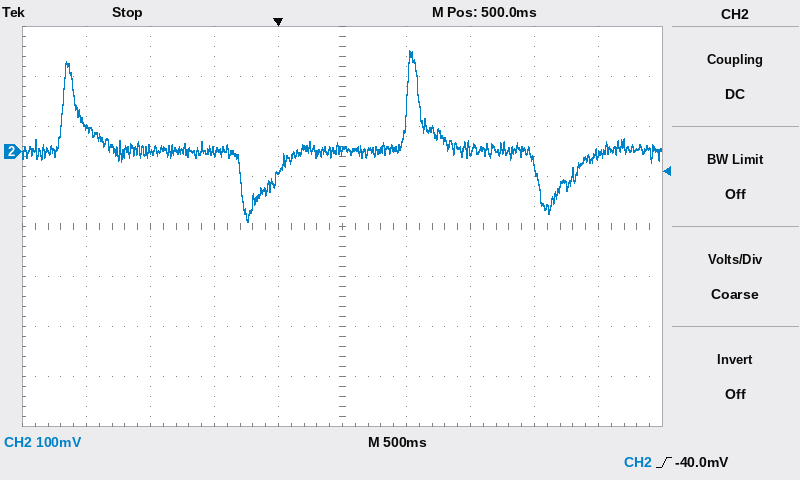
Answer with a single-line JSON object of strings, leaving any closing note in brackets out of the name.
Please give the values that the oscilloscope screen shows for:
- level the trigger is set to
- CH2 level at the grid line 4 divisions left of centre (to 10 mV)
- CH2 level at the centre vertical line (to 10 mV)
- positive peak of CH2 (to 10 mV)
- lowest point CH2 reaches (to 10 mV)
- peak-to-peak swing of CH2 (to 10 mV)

{"level the trigger is set to": "-40.0 mV", "CH2 level at the grid line 4 divisions left of centre": "50 mV", "CH2 level at the centre vertical line": "0 mV", "positive peak of CH2": "200 mV", "lowest point CH2 reaches": "-140 mV", "peak-to-peak swing of CH2": "340 mV"}
